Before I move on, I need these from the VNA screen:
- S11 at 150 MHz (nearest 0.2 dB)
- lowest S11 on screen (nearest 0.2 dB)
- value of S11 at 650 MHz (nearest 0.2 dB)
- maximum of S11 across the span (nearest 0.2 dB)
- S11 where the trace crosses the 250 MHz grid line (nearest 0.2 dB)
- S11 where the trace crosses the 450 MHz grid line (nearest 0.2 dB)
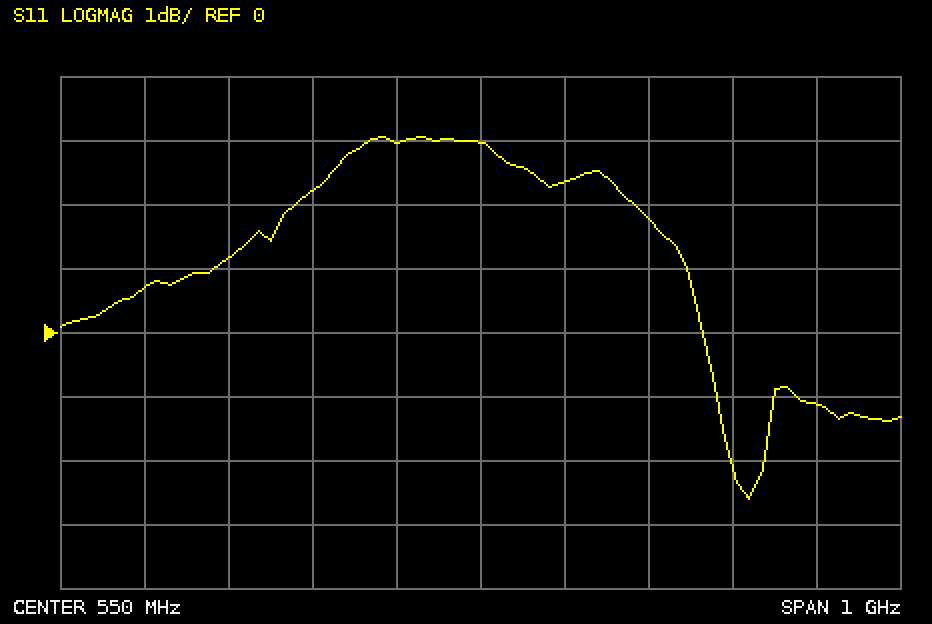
0.8 dB
-2.6 dB
2.4 dB
3.0 dB
1.2 dB
3.0 dB
